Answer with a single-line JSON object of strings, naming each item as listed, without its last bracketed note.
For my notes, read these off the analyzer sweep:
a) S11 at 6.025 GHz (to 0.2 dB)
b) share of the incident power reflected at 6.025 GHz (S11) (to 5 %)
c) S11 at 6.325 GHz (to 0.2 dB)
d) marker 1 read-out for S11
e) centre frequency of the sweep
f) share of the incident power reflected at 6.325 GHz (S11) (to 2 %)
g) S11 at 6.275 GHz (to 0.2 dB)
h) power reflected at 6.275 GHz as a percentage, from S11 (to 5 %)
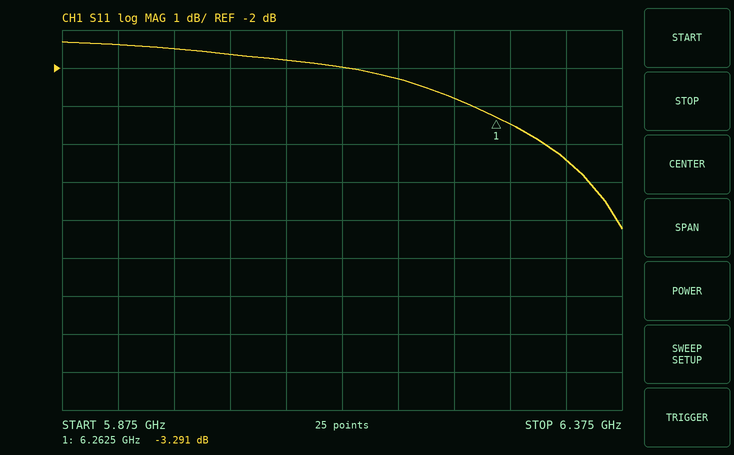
{"S11 at 6.025 GHz": "-1.6 dB", "share of the incident power reflected at 6.025 GHz (S11)": "70 %", "S11 at 6.325 GHz": "-4.4 dB", "marker 1 read-out for S11": "-3.291 dB", "centre frequency of the sweep": "6.125 GHz", "share of the incident power reflected at 6.325 GHz (S11)": "36 %", "S11 at 6.275 GHz": "-3.4 dB", "power reflected at 6.275 GHz as a percentage, from S11": "45 %"}
